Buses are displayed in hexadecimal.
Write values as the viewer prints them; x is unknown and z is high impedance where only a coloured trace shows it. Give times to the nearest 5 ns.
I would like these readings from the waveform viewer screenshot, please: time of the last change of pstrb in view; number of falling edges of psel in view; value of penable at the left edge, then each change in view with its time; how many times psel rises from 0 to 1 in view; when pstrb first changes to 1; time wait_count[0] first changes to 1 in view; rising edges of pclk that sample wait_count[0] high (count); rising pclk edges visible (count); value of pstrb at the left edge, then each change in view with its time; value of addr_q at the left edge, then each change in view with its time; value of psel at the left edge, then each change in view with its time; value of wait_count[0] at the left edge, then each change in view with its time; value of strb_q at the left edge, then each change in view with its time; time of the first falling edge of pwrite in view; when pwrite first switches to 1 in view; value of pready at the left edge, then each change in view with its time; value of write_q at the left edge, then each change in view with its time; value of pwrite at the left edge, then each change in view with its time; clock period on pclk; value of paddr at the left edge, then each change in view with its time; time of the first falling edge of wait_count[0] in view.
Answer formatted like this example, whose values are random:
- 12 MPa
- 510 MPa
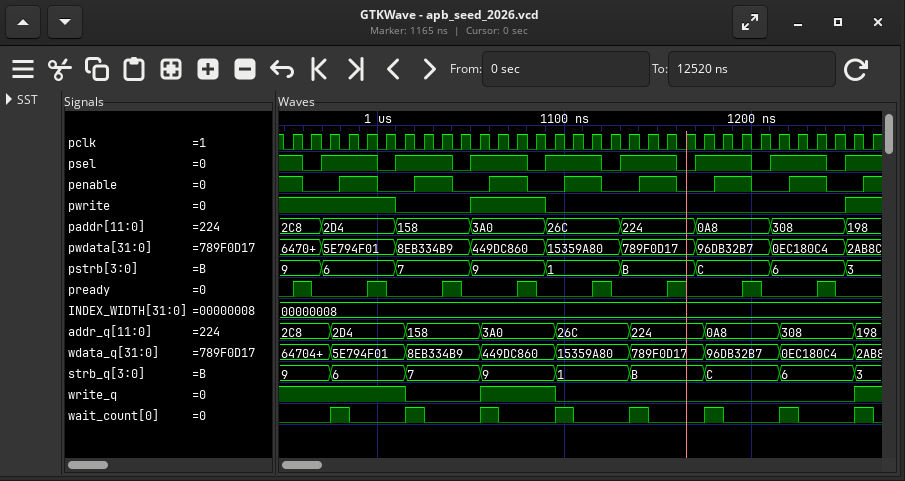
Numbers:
- 1250 ns
- 8
- 1, 0 at 960 ns, 1 at 980 ns, 0 at 1000 ns, 1 at 1020 ns, 0 at 1040 ns, 1 at 1060 ns, 0 at 1080 ns, 1 at 1100 ns, 0 at 1120 ns, 1 at 1140 ns, 0 at 1160 ns, 1 at 1180 ns, 0 at 1200 ns, 1 at 1220 ns, 0 at 1240 ns, 1 at 1260 ns
- 8
- 1090 ns
- 975 ns
- 8
- 32
- 9, 6 at 970 ns, 7 at 1010 ns, 9 at 1050 ns, 1 at 1090 ns, B at 1130 ns, C at 1170 ns, 6 at 1210 ns, 3 at 1250 ns
- 2C8, 2D4 at 975 ns, 158 at 1015 ns, 3A0 at 1055 ns, 26C at 1095 ns, 224 at 1135 ns, 0A8 at 1175 ns, 308 at 1215 ns, 198 at 1255 ns
- 1, 0 at 960 ns, 1 at 970 ns, 0 at 1000 ns, 1 at 1010 ns, 0 at 1040 ns, 1 at 1050 ns, 0 at 1080 ns, 1 at 1090 ns, 0 at 1120 ns, 1 at 1130 ns, 0 at 1160 ns, 1 at 1170 ns, 0 at 1200 ns, 1 at 1210 ns, 0 at 1240 ns, 1 at 1250 ns
- 0, 1 at 975 ns, 0 at 985 ns, 1 at 1015 ns, 0 at 1025 ns, 1 at 1055 ns, 0 at 1065 ns, 1 at 1095 ns, 0 at 1105 ns, 1 at 1135 ns, 0 at 1145 ns, 1 at 1175 ns, 0 at 1185 ns, 1 at 1215 ns, 0 at 1225 ns, 1 at 1255 ns, 0 at 1265 ns
- 9, 6 at 975 ns, 7 at 1015 ns, 9 at 1055 ns, 1 at 1095 ns, B at 1135 ns, C at 1175 ns, 6 at 1215 ns, 3 at 1255 ns
- 1010 ns
- 1050 ns
- 0, 1 at 955 ns, 0 at 965 ns, 1 at 995 ns, 0 at 1005 ns, 1 at 1035 ns, 0 at 1045 ns, 1 at 1075 ns, 0 at 1085 ns, 1 at 1115 ns, 0 at 1125 ns, 1 at 1155 ns, 0 at 1165 ns, 1 at 1195 ns, 0 at 1205 ns, 1 at 1235 ns, 0 at 1245 ns
- 1, 0 at 1015 ns, 1 at 1055 ns, 0 at 1095 ns, 1 at 1255 ns
- 1, 0 at 1010 ns, 1 at 1050 ns, 0 at 1090 ns, 1 at 1250 ns
- 10 ns
- 2C8, 2D4 at 970 ns, 158 at 1010 ns, 3A0 at 1050 ns, 26C at 1090 ns, 224 at 1130 ns, 0A8 at 1170 ns, 308 at 1210 ns, 198 at 1250 ns
- 985 ns
